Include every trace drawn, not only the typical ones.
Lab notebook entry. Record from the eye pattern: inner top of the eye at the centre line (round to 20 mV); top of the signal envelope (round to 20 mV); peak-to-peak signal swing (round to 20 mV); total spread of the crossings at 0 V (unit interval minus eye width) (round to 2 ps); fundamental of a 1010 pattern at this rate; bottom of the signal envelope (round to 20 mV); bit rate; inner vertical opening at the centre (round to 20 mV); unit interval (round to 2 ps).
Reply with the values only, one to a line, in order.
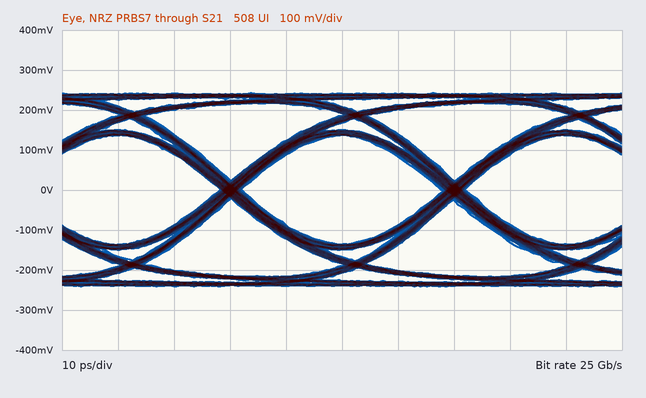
140 mV
240 mV
480 mV
4 ps
12.5 GHz
-240 mV
25 Gb/s
280 mV
40 ps
